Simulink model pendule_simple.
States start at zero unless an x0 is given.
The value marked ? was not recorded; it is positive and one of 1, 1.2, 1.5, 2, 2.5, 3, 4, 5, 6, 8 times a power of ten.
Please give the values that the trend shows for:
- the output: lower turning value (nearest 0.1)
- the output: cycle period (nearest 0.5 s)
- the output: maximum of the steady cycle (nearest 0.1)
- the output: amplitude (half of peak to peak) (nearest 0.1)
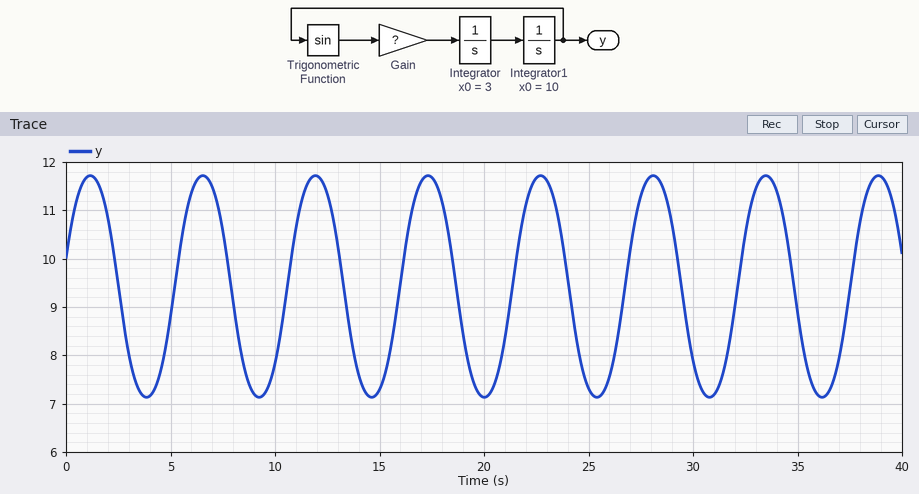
7.1
5.5 s
11.7
2.3
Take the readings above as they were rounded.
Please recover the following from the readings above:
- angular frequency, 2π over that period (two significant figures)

1.1 rad/s
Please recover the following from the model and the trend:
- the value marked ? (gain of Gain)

3
